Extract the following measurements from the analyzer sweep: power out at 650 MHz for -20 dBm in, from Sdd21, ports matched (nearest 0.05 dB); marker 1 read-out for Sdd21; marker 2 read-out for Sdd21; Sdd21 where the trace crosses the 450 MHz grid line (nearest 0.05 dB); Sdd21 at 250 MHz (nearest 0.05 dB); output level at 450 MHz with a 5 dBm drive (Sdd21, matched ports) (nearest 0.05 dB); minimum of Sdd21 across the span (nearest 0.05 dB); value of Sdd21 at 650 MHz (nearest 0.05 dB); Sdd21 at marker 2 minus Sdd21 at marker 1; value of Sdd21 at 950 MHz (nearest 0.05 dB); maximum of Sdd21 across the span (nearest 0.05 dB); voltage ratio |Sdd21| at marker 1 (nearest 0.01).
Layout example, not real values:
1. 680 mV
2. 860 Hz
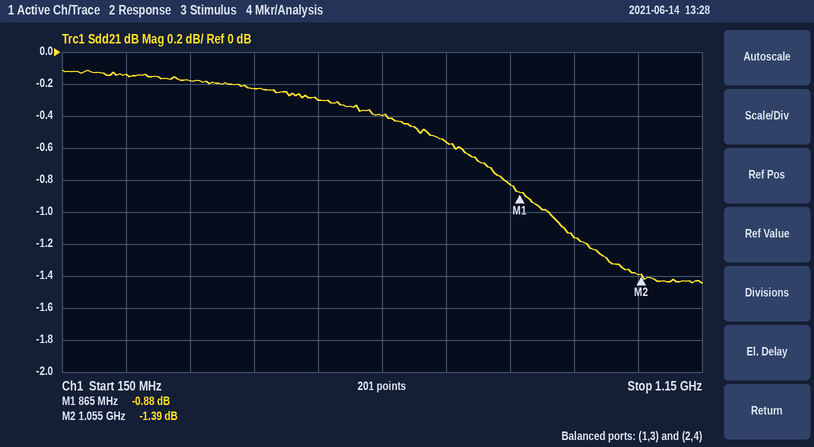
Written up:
1. -20.40 dBm
2. -0.88 dB
3. -1.39 dB
4. -0.25 dB
5. -0.15 dB
6. 4.75 dBm
7. -1.45 dB
8. -0.40 dB
9. -0.51 dB
10. -1.15 dB
11. -0.10 dB
12. 0.90
